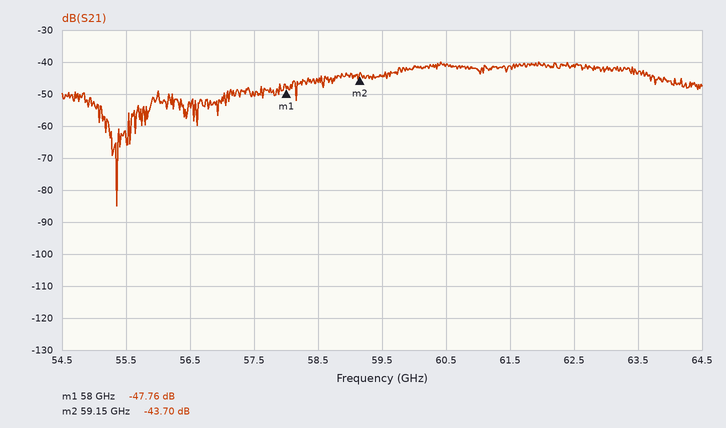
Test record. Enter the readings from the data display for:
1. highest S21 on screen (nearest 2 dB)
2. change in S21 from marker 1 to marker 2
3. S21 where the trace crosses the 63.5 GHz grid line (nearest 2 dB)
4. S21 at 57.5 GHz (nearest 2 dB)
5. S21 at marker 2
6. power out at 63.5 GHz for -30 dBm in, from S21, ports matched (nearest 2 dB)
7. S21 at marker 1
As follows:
-40 dB
4.06 dB
-44 dB
-50 dB
-43.70 dB
-74 dBm
-47.76 dB
